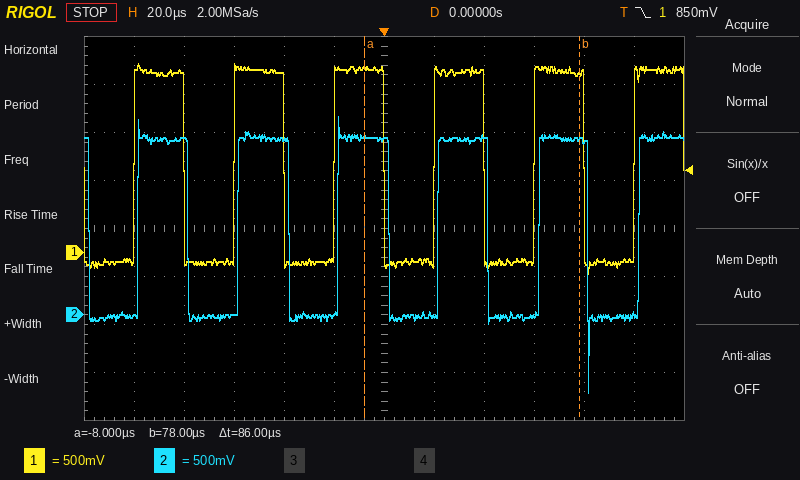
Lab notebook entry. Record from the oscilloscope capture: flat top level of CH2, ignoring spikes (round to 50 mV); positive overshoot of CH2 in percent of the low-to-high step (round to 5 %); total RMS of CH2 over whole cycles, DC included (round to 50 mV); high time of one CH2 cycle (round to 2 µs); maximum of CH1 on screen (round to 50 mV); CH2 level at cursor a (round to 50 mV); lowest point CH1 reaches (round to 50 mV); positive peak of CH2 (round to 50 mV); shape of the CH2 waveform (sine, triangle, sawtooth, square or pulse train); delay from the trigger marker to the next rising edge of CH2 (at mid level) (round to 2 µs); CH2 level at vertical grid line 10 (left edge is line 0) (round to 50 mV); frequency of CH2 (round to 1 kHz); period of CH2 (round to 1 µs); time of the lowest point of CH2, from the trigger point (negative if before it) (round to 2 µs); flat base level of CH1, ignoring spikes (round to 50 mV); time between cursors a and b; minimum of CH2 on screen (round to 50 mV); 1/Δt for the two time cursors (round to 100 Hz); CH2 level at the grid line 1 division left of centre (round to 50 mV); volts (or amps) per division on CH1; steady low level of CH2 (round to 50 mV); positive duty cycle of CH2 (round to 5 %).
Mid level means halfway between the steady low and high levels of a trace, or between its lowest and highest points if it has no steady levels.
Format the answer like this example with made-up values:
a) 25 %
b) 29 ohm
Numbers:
a) 1.85 V
b) 10 %
c) 1.30 V
d) 20 µs
e) 1.95 V
f) 1.85 V
g) -200 mV
h) 2.05 V
i) square
j) 22 µs
k) 1.80 V
l) 25 kHz
m) 40 µs
n) +82 µs
o) -100 mV
p) 86 µs
q) -800 mV
r) 11.6 kHz
s) 0 mV
t) 500 mV
u) 0 mV
v) 50 %
